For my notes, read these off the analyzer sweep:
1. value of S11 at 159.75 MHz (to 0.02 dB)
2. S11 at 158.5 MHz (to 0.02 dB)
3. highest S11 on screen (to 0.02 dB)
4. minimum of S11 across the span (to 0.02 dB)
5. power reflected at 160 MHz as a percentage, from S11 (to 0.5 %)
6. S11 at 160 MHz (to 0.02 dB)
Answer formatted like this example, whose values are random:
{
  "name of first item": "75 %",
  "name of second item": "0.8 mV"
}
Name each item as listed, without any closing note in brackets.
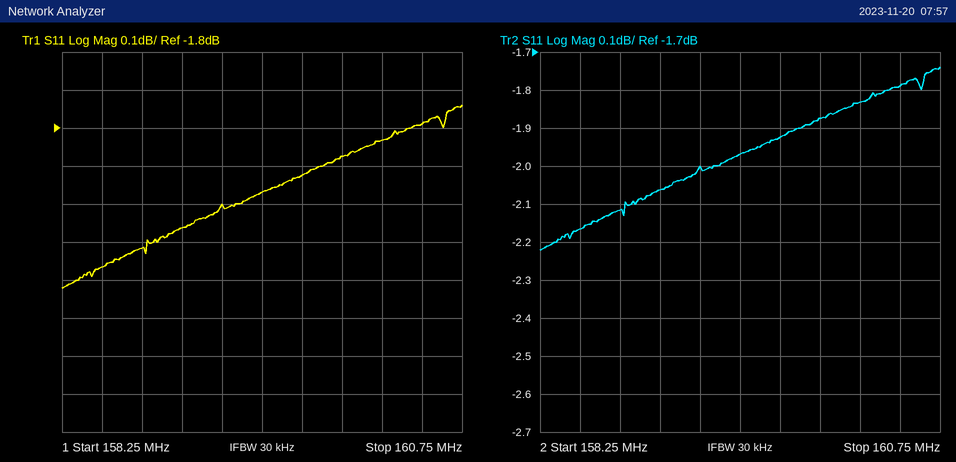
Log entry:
{
  "value of S11 at 159.75 MHz": "-1.92 dB",
  "S11 at 158.5 MHz": "-2.16 dB",
  "highest S11 on screen": "-1.74 dB",
  "minimum of S11 across the span": "-2.22 dB",
  "power reflected at 160 MHz as a percentage, from S11": "65.0 %",
  "S11 at 160 MHz": "-1.88 dB"
}
